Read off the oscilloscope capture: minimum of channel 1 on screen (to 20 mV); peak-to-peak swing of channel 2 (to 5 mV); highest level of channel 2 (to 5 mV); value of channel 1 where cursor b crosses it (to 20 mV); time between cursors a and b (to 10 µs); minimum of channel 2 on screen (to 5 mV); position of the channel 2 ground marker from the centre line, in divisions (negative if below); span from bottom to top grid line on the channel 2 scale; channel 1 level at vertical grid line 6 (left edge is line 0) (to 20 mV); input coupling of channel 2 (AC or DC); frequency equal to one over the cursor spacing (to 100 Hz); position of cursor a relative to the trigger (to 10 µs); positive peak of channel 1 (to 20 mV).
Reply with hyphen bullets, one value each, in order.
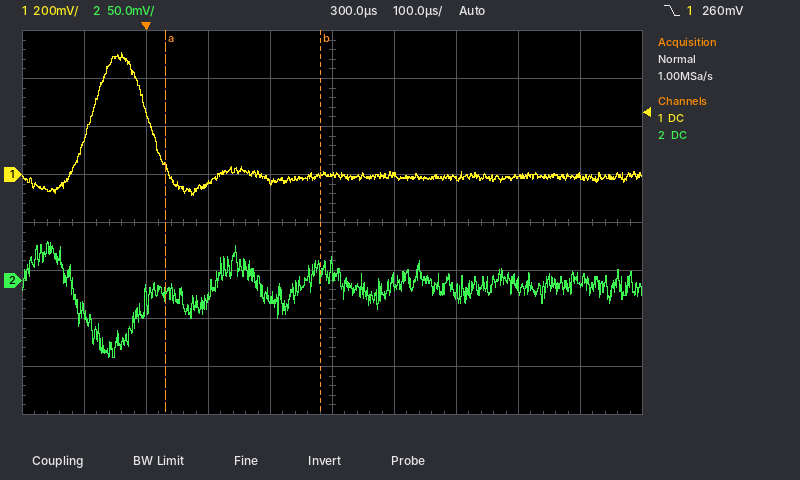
- -80 mV
- 120 mV
- 40 mV
- 0 mV
- 250 µs
- -80 mV
- -1.2 div
- 400 mV
- 0 mV
- DC
- 4.0 kHz
- +30 µs
- 500 mV
